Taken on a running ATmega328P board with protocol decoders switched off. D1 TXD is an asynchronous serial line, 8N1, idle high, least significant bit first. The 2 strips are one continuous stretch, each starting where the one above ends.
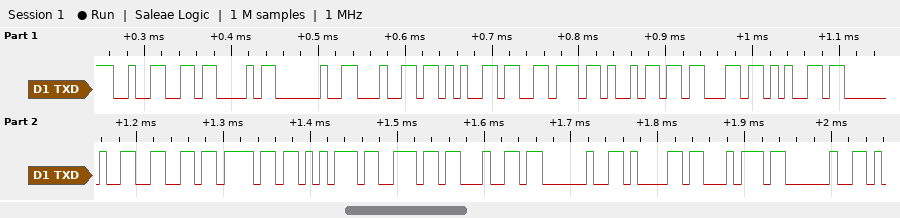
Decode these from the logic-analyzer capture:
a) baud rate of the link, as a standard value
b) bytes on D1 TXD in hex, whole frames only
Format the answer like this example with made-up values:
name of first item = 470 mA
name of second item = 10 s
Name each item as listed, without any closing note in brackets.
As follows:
baud rate of the link, as a standard value = 115200 baud
bytes on D1 TXD in hex, whole frames only = 32 43 20 64 65 76 69 63 65 20 66 6F 75 6E 64 20 61 74 20
